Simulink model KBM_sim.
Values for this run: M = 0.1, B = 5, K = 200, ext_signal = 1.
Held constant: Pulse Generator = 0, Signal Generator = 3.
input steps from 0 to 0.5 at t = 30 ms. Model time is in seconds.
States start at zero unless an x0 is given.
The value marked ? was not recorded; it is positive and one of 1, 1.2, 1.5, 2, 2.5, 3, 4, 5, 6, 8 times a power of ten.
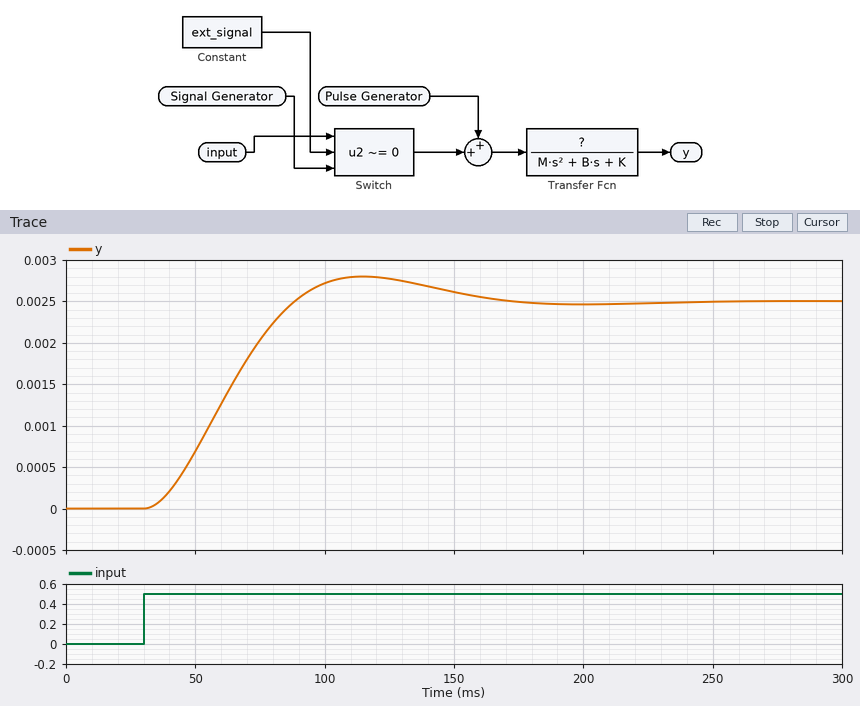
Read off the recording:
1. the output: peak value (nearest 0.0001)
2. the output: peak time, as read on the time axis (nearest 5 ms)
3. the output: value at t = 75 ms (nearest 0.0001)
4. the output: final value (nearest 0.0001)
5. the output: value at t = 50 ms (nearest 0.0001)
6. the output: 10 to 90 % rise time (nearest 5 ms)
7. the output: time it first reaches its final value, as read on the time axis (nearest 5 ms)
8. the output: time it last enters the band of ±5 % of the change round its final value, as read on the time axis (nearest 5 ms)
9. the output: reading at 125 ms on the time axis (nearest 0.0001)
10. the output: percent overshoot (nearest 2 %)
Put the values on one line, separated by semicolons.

0.0028; 115 ms; 0.0020; 0.0025; 0.0007; 40 ms; 90 ms; 150 ms; 0.0028; 12 %
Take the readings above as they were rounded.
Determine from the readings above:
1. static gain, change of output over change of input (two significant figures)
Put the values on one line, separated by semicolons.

0.0050
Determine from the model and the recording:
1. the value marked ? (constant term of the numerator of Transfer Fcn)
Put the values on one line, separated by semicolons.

1
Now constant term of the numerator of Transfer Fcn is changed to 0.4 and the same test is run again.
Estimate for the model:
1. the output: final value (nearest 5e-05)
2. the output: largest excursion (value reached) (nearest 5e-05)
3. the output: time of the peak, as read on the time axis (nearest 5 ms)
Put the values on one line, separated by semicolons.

0.00100; 0.00110; 115 ms
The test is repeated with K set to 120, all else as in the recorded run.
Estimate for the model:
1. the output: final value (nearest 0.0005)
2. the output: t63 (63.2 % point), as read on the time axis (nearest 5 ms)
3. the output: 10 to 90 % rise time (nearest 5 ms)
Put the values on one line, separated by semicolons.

0.0040; 80 ms; 65 ms
